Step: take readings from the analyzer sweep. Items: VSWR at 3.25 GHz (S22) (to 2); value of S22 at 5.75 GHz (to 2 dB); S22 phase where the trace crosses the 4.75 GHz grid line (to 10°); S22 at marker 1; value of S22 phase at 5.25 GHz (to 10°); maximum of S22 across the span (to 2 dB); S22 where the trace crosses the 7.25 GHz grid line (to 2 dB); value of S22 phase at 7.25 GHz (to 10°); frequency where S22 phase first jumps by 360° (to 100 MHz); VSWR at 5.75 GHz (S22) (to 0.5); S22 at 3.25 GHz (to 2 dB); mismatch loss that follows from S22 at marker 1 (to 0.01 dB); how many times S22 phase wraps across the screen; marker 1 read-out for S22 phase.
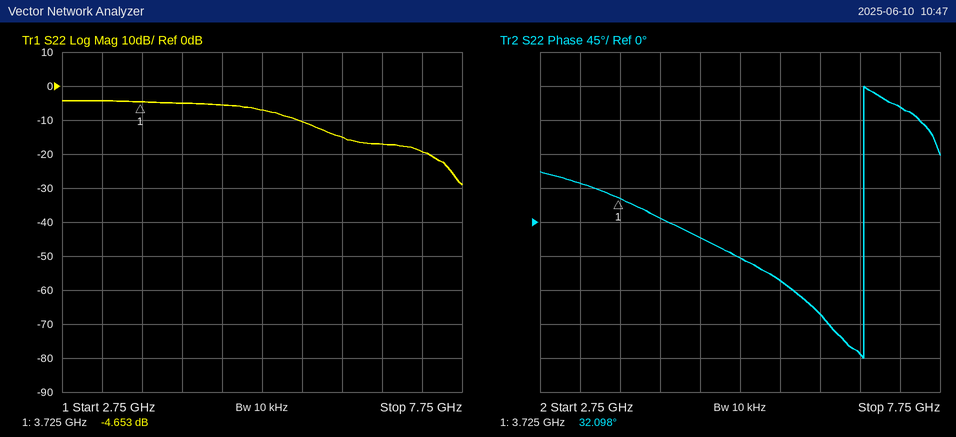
4
-10 dB
-20°
-4.653 dB
-50°
-4 dB
-20 dB
150°
6.8 GHz
2.0
-4 dB
1.82 dB
1
32.098°
